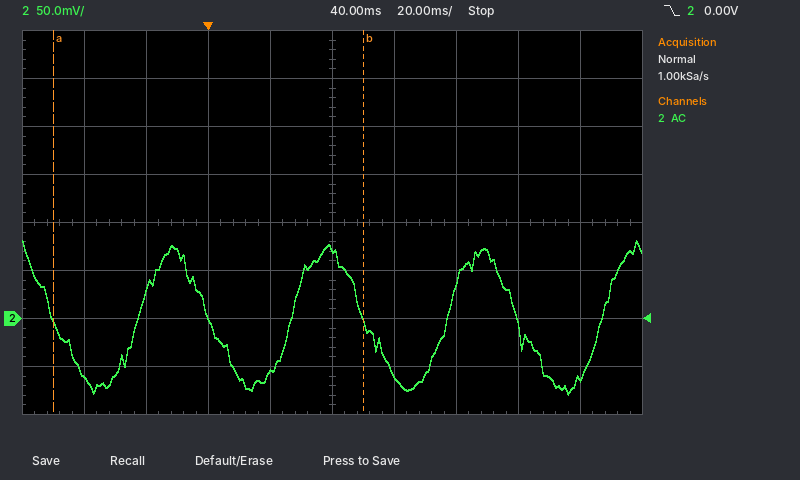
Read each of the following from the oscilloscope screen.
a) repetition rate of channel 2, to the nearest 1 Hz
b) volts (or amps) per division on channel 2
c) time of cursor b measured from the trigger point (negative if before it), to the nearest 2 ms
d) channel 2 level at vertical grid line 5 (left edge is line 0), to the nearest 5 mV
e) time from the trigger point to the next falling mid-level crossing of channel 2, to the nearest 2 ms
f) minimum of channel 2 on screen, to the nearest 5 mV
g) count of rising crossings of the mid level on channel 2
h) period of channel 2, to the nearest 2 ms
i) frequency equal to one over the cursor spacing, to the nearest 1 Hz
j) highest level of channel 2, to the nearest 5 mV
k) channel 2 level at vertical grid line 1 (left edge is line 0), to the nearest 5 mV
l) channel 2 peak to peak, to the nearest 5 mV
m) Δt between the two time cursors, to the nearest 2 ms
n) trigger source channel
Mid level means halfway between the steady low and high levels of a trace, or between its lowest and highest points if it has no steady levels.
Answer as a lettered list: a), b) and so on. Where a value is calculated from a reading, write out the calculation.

a) 1 / 50 ms ≈ 20 Hz
b) 50 mV
c) +50 ms
d) 75 mV
e) 50 ms
f) -80 mV
g) 4
h) 50 ms
i) 1 / 100 ms ≈ 10 Hz
j) 80 mV
k) -60 mV
l) 80 mV − (-80 mV) = 160 mV
m) 100 ms
n) channel 2
